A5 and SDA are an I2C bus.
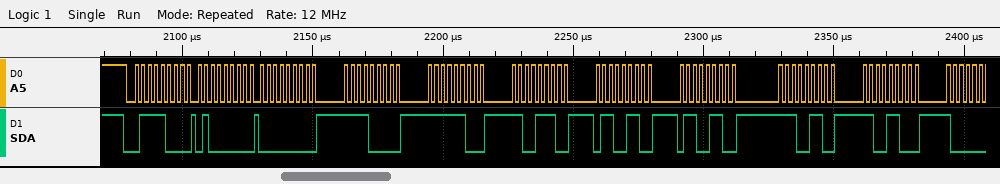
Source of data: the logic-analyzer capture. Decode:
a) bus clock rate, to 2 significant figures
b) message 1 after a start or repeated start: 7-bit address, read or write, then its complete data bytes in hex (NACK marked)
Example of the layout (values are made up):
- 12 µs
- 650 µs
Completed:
- 400 kHz
- 0x3C write: 40 00 F0 FC CE 66 66 E6 CC
